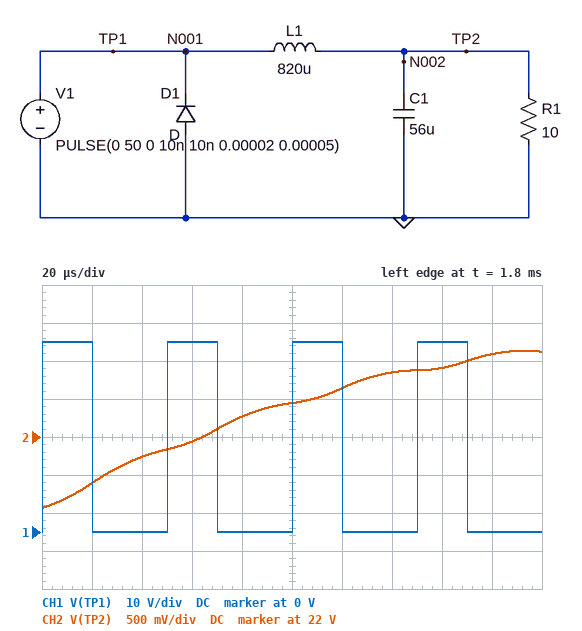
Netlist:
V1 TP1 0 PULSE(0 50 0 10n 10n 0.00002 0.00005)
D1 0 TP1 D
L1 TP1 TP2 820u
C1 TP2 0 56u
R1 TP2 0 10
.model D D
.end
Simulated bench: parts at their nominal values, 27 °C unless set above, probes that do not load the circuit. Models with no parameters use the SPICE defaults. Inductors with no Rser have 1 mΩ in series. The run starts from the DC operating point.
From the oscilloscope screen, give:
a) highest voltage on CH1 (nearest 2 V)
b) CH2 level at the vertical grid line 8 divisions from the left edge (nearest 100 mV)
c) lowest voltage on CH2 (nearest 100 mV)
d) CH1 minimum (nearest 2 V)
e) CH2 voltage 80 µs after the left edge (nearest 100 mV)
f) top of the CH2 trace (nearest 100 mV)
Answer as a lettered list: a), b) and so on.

a) 50 V
b) 22.9 V
c) 21.1 V
d) 0 V
e) 22.3 V
f) 23.1 V
